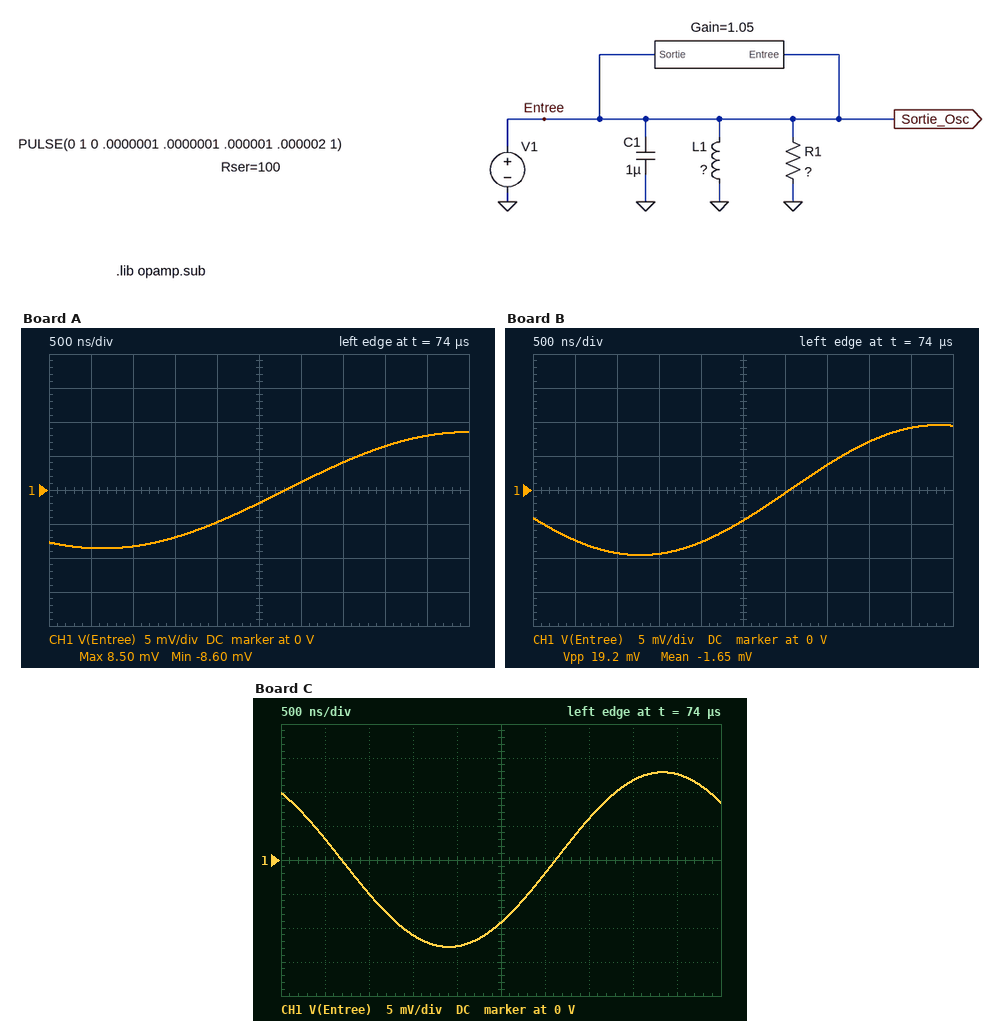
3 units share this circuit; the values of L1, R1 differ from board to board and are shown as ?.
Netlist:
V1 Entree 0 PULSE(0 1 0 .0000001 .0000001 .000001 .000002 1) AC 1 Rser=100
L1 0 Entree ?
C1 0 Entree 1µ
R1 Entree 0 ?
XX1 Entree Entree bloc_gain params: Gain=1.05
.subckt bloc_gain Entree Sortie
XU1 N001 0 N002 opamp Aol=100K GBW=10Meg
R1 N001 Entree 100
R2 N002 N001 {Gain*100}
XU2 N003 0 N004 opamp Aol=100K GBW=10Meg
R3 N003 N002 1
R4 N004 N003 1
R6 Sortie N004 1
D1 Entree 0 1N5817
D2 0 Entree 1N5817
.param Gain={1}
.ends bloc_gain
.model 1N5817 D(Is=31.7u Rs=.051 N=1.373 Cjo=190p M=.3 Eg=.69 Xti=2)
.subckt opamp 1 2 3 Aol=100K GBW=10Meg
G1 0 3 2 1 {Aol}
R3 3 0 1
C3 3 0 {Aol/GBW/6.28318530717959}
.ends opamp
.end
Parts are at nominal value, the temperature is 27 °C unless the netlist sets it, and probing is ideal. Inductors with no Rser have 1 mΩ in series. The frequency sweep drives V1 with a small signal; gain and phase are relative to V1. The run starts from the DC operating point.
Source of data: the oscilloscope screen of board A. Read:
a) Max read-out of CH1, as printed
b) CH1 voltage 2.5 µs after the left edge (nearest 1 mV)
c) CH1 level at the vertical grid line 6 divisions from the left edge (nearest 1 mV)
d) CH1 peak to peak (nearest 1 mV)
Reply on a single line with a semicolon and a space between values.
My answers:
8.50 mV; -2 mV; 1 mV; 17 mV
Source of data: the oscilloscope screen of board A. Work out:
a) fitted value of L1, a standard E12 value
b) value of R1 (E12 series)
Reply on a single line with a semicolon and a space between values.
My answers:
1.8 µH; 33 Ω
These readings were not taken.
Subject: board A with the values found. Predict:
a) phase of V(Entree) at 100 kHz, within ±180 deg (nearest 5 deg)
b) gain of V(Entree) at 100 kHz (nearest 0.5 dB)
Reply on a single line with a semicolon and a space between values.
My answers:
90 deg; -26.5 dB
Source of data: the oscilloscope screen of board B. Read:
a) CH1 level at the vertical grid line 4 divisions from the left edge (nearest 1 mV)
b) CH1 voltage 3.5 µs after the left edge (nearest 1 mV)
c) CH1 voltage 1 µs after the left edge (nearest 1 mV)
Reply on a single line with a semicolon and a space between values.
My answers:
-8 mV; 4 mV; -9 mV
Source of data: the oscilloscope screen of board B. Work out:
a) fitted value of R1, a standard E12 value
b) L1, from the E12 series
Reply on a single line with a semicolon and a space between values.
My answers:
39 Ω; 1.2 µH
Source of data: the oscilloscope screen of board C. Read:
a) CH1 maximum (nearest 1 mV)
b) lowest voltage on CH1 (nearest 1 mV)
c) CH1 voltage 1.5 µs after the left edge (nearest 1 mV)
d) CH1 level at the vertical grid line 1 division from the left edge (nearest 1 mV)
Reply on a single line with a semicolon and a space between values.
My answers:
13 mV; -13 mV; -11 mV; 3 mV
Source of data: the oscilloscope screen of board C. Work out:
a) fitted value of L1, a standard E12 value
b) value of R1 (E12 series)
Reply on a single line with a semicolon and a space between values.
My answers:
560 nH; 82 Ω
